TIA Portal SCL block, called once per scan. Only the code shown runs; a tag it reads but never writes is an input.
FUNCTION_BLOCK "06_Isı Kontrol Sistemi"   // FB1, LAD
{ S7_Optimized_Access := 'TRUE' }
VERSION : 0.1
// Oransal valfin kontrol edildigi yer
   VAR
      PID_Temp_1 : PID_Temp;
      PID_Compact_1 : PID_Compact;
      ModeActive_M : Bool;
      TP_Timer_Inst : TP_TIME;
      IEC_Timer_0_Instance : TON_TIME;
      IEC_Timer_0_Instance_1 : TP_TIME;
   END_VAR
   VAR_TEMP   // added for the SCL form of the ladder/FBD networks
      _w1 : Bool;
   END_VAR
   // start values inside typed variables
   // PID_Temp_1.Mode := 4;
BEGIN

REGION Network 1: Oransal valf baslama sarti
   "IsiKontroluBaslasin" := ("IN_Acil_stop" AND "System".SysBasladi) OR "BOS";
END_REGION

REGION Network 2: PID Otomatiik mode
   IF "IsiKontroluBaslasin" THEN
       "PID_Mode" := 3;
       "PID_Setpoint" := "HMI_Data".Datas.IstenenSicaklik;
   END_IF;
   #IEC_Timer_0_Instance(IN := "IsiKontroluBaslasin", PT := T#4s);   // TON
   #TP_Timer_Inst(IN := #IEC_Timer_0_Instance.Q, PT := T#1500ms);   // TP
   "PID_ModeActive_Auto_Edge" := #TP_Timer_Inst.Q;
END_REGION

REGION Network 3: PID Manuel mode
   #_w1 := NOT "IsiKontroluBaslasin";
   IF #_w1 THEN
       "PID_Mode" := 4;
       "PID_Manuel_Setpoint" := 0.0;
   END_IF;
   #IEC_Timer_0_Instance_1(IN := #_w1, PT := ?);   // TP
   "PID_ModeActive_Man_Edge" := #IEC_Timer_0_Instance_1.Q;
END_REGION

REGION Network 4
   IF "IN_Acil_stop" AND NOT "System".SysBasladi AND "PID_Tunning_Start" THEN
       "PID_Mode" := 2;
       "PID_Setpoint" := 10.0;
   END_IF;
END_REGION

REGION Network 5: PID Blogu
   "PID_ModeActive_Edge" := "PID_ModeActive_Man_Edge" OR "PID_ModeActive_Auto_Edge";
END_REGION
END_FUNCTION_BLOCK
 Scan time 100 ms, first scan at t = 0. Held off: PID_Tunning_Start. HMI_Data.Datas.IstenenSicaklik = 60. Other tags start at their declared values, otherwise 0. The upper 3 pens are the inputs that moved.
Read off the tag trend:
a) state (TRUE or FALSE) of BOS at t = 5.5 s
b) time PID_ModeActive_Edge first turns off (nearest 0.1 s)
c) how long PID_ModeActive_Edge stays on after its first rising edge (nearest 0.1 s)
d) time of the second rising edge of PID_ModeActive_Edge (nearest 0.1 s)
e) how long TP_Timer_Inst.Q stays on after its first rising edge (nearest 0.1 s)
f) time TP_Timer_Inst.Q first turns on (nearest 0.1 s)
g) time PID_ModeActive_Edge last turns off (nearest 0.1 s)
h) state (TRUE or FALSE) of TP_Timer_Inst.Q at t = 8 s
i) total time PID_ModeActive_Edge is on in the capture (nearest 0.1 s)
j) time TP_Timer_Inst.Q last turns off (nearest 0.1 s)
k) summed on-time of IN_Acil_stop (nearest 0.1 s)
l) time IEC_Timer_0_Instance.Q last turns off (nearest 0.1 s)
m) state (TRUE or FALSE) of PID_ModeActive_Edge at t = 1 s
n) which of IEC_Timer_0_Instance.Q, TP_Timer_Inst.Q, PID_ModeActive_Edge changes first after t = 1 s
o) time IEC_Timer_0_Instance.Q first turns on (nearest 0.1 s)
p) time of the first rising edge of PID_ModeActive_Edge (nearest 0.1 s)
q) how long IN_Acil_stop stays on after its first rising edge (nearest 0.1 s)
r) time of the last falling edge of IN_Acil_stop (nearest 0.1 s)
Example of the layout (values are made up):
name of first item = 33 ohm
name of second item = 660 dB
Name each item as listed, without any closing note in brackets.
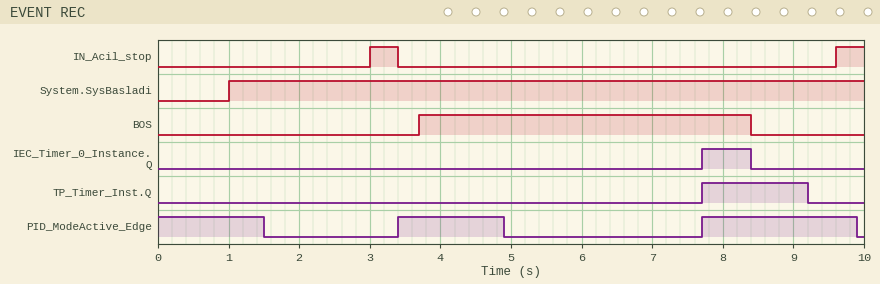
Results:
state (TRUE or FALSE) of BOS at t = 5.5 s = TRUE
time PID_ModeActive_Edge first turns off = 1.5 s
how long PID_ModeActive_Edge stays on after its first rising edge = 1.5 s
time of the second rising edge of PID_ModeActive_Edge = 7.7 s
how long TP_Timer_Inst.Q stays on after its first rising edge = 1.5 s
time TP_Timer_Inst.Q first turns on = 7.7 s
time PID_ModeActive_Edge last turns off = 9.9 s
state (TRUE or FALSE) of TP_Timer_Inst.Q at t = 8 s = TRUE
total time PID_ModeActive_Edge is on in the capture = 5.2 s
time TP_Timer_Inst.Q last turns off = 9.2 s
summed on-time of IN_Acil_stop = 0.8 s
time IEC_Timer_0_Instance.Q last turns off = 8.4 s
state (TRUE or FALSE) of PID_ModeActive_Edge at t = 1 s = TRUE
which of IEC_Timer_0_Instance.Q, TP_Timer_Inst.Q, PID_ModeActive_Edge changes first after t = 1 s = PID_ModeActive_Edge
time IEC_Timer_0_Instance.Q first turns on = 7.7 s
time of the first rising edge of PID_ModeActive_Edge = 3.4 s
how long IN_Acil_stop stays on after its first rising edge = 0.4 s
time of the last falling edge of IN_Acil_stop = 3.4 s
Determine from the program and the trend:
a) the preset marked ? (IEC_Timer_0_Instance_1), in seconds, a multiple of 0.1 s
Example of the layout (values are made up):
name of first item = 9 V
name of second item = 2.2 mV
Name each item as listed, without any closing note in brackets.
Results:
the preset marked ? (IEC_Timer_0_Instance_1), in seconds, a multiple of 0.1 s = 1.5 s
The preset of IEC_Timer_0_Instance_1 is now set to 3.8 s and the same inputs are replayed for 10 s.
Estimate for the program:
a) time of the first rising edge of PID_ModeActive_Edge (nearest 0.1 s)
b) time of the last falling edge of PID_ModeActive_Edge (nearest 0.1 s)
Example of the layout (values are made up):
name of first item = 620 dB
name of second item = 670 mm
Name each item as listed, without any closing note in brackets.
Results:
time of the first rising edge of PID_ModeActive_Edge = 7.7 s
time of the last falling edge of PID_ModeActive_Edge = 3.8 s
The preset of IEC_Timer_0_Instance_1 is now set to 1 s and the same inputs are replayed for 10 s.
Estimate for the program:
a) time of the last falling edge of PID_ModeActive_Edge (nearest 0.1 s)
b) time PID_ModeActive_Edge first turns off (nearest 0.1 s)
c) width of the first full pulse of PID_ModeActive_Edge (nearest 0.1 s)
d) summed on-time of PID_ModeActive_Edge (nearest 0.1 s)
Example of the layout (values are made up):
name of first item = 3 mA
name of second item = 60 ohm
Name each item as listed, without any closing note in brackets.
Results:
time of the last falling edge of PID_ModeActive_Edge = 9.4 s
time PID_ModeActive_Edge first turns off = 1.0 s
width of the first full pulse of PID_ModeActive_Edge = 1.0 s
summed on-time of PID_ModeActive_Edge = 3.7 s
